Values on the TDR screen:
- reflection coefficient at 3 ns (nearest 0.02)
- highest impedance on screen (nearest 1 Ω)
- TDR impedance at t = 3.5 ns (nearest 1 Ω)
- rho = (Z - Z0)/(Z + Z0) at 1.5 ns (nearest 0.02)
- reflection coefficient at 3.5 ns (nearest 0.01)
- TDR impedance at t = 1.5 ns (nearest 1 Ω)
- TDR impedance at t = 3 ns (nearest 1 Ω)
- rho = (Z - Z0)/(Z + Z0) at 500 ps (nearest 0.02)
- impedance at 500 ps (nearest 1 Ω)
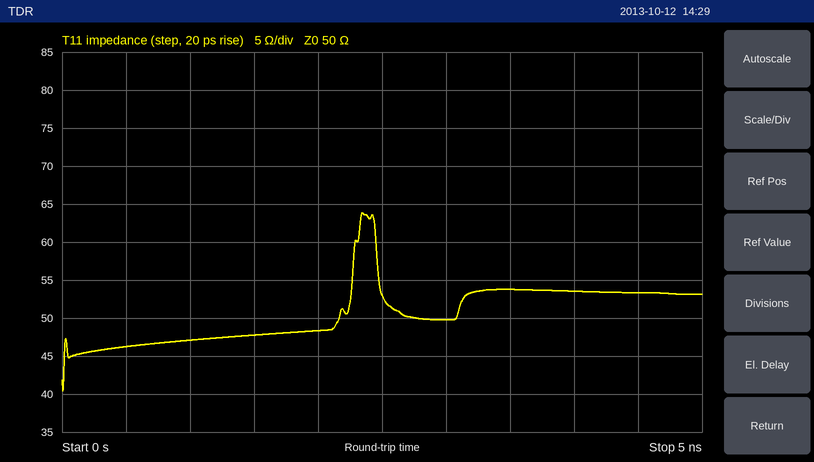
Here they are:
0.00
64 Ω
54 Ω
-0.02
+0.04
48 Ω
50 Ω
-0.04
46 Ω
